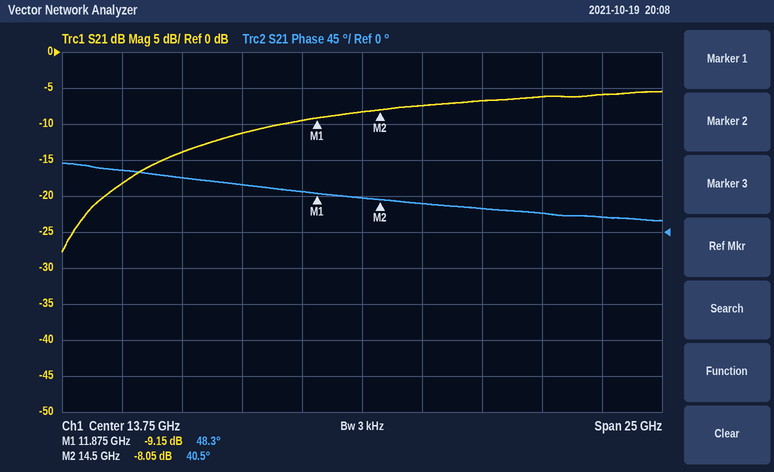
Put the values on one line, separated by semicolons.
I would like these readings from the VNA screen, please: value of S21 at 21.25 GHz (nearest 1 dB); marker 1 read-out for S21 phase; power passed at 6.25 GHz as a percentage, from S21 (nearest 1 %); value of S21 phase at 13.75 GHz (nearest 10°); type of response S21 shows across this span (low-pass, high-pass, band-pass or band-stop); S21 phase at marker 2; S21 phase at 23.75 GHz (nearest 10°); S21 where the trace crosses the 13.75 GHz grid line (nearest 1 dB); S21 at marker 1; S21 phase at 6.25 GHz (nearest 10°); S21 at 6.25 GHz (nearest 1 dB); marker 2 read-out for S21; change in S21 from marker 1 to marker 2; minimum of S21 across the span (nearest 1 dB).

-6 dB; 48.3°; 4 %; 40°; high-pass; 40.5°; 20°; -8 dB; -9.15 dB; 70°; -14 dB; -8.05 dB; 1.10 dB; -28 dB
